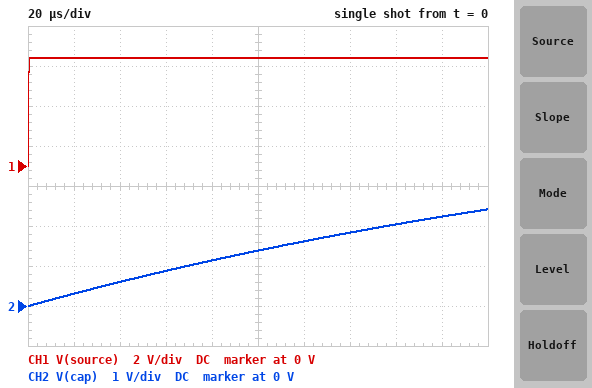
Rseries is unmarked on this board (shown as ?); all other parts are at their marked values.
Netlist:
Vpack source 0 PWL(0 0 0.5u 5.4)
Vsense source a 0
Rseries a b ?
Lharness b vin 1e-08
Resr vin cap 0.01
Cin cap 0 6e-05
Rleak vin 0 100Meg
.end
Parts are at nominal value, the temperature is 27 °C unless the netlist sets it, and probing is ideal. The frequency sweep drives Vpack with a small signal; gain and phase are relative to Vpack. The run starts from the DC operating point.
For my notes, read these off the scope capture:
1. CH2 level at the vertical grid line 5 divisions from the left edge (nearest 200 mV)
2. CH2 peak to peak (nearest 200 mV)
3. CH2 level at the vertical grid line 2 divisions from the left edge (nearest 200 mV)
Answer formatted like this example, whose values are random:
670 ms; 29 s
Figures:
1.4 V; 2.4 V; 600 mV
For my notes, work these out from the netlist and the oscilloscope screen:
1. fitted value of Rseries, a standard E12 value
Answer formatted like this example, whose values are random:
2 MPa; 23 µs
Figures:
5.6 Ω
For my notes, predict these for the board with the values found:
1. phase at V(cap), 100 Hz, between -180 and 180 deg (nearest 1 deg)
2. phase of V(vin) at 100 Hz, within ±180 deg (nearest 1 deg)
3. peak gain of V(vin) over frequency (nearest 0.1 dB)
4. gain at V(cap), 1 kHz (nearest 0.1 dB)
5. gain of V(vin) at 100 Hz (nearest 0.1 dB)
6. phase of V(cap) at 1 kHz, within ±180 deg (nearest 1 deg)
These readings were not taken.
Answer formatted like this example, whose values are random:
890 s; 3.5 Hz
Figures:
-12 deg; -12 deg; 0 dB; -7.4 dB; -0.2 dB; -65 deg
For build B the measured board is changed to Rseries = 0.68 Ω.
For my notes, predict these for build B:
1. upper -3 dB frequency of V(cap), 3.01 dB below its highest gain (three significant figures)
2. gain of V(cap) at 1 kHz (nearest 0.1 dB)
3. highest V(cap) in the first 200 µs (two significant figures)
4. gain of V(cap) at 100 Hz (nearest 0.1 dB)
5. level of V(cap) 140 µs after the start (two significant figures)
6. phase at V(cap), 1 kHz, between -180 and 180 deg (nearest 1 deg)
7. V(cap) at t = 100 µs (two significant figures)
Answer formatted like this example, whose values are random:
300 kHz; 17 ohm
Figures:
3.85 kHz; -0.3 dB; 5.4 V; 0 dB; 5.2 V; -15 deg; 4.9 V
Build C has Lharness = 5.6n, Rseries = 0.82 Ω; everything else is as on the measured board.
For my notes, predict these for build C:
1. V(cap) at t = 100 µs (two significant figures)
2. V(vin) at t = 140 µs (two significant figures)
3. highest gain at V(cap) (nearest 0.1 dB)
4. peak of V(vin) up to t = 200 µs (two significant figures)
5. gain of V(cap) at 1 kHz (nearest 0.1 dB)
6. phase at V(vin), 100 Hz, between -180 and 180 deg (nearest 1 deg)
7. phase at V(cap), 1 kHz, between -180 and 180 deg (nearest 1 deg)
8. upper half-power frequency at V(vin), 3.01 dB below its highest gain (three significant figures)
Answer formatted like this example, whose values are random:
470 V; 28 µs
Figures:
4.7 V; 5.1 V; 0 dB; 5.3 V; -0.4 dB; -2 deg; -17 deg; 3.20 kHz
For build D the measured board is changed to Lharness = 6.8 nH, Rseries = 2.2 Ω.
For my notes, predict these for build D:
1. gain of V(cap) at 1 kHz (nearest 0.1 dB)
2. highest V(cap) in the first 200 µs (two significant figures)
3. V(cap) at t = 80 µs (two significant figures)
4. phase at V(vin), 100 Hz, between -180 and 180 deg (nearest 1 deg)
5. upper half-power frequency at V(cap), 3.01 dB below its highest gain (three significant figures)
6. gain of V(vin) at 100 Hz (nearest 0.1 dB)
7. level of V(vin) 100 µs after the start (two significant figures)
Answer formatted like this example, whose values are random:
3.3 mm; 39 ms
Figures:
-2.3 dB; 4.2 V; 2.4 V; -5 deg; 1.20 kHz; 0 dB; 2.9 V
